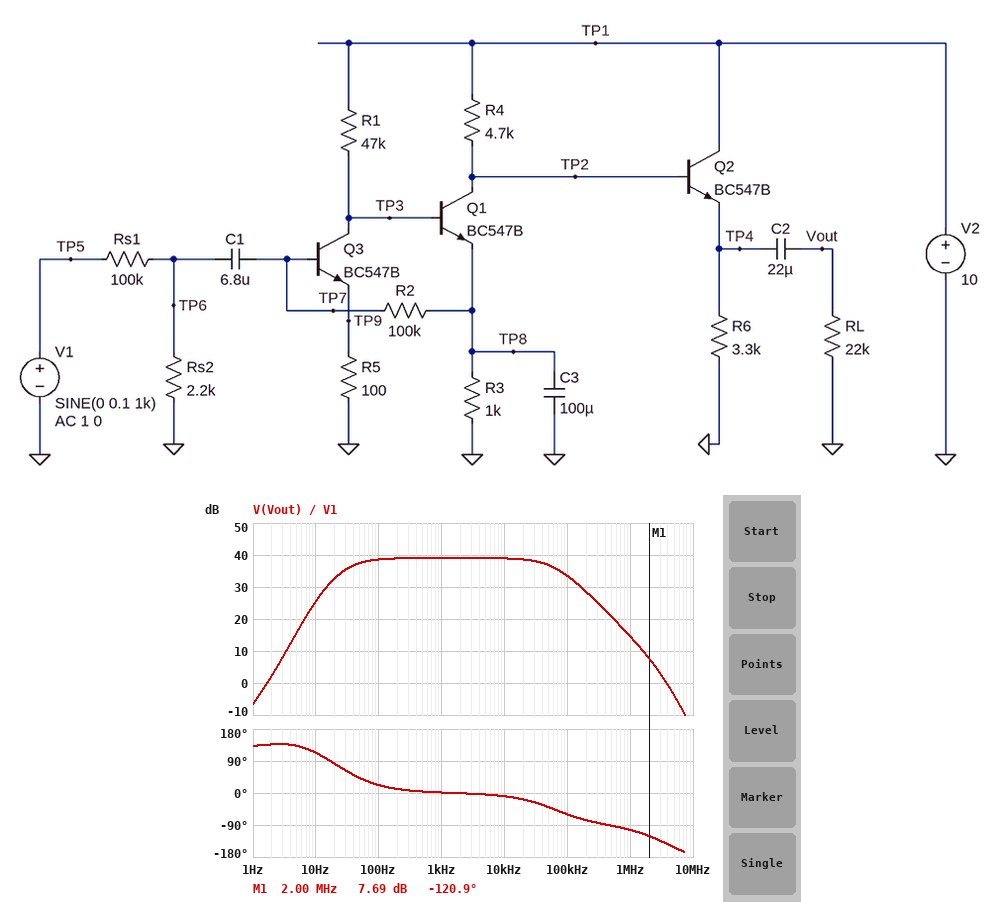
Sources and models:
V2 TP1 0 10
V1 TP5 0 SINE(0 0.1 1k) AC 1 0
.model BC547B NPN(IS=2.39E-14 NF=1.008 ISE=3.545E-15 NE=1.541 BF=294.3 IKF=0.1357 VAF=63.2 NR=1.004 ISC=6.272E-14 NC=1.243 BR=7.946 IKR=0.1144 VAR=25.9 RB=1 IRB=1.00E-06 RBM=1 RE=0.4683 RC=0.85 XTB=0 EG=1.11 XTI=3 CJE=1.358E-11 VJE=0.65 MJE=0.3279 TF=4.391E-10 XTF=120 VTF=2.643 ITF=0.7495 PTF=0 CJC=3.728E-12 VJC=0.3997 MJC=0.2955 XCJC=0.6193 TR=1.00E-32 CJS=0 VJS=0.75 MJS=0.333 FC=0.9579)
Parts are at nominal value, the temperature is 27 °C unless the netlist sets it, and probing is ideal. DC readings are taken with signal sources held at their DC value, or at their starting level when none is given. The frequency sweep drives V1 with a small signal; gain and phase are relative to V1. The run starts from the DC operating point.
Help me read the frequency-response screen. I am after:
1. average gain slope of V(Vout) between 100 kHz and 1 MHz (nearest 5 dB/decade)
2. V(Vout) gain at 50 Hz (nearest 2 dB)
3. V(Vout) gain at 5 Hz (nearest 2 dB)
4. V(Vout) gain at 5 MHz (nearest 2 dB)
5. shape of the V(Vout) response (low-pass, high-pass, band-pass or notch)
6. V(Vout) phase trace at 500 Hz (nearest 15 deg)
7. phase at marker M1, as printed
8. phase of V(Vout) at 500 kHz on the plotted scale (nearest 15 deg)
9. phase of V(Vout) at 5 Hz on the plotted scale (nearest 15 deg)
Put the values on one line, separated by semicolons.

-20 dB/decade; 38 dB; 16 dB; -4 dB; band-pass; 0 deg; -120.9 deg; -90 deg; 135 deg
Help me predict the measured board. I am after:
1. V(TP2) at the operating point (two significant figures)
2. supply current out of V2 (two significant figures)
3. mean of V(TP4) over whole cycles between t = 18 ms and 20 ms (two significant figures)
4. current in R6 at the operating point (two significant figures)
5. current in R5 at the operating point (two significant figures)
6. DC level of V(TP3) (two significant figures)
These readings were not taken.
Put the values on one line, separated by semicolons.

6.8 V; 2.7 mA; 6.2 V; 1.9 mA; 180 µA; 1.3 V
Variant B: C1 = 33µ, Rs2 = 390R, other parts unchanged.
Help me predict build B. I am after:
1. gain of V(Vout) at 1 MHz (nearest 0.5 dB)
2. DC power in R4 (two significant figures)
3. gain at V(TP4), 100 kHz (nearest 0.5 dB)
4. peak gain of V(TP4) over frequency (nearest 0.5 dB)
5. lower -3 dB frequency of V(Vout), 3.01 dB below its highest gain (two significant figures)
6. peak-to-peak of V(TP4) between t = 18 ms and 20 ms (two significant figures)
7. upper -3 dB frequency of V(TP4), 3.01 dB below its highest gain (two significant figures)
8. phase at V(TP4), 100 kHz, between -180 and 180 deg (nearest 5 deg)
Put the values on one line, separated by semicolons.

1.0 dB; 2.2 mW; 19.5 dB; 24.5 dB; 12 Hz; 3.3 V; 67 kHz; -55 deg
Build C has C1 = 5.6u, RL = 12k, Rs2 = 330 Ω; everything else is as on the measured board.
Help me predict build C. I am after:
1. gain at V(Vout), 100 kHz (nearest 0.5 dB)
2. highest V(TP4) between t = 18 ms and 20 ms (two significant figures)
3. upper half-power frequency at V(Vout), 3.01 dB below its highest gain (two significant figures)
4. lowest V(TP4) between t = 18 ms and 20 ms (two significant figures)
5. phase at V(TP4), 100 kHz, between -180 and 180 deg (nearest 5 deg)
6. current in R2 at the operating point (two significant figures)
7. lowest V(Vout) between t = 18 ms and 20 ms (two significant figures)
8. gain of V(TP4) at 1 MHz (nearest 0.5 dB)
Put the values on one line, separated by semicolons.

18.0 dB; 7.5 V; 150 Hz; 4.7 V; -55 deg; 640 nA; -1.4 V; -0.5 dB
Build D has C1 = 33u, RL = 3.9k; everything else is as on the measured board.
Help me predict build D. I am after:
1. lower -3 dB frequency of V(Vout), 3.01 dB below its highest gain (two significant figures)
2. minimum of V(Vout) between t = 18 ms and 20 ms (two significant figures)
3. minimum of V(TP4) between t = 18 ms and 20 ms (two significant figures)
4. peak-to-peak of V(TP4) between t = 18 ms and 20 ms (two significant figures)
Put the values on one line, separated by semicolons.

39 Hz; -3.4 V; 2.8 V; 6.4 V
